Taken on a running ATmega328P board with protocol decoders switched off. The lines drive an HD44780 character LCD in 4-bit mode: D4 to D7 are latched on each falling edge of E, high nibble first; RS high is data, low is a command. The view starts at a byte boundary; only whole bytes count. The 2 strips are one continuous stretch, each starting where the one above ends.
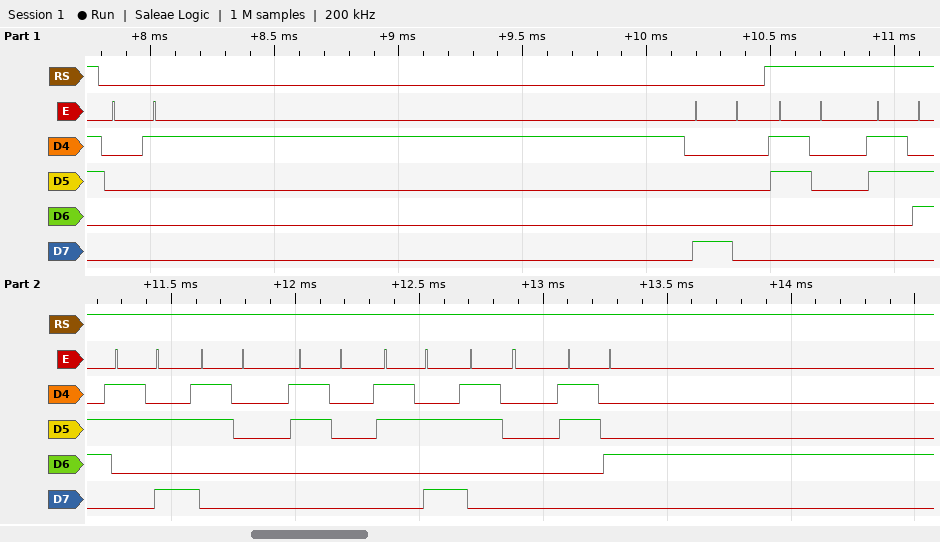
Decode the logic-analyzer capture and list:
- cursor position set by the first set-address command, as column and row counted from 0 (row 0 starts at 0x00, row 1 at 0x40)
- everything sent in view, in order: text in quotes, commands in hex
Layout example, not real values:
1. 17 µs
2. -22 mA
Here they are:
1. column 0, row 0
2. 0x01 0x80 "06:00:04"
